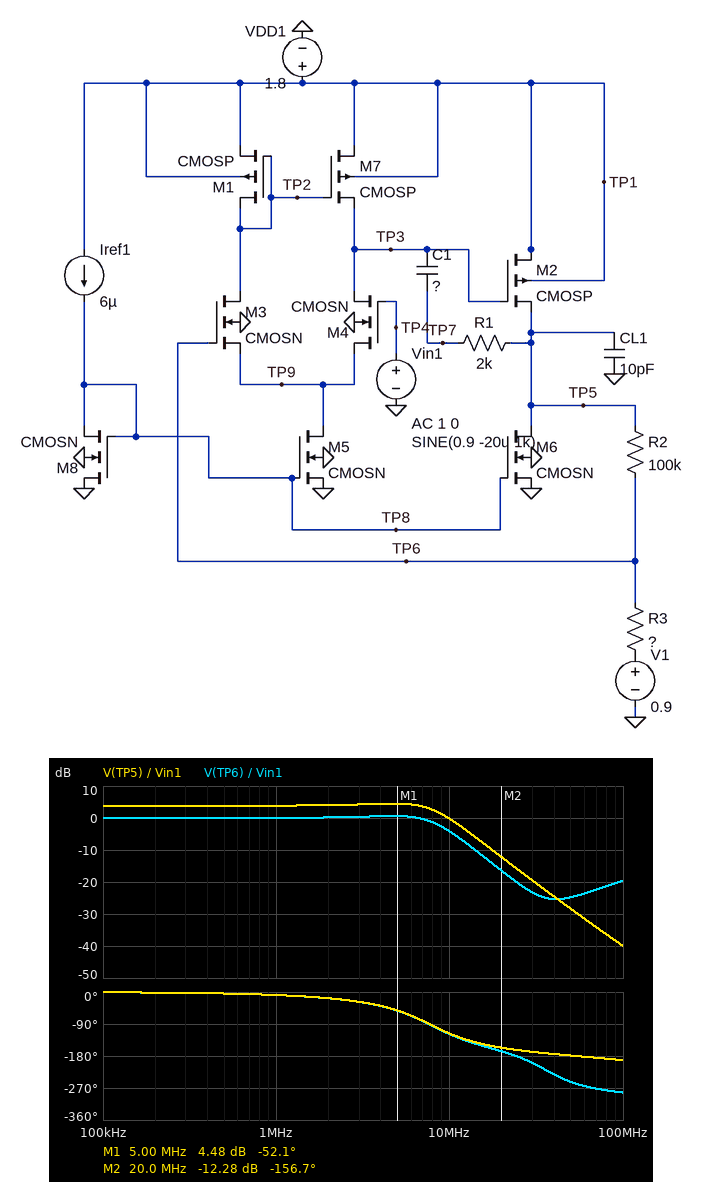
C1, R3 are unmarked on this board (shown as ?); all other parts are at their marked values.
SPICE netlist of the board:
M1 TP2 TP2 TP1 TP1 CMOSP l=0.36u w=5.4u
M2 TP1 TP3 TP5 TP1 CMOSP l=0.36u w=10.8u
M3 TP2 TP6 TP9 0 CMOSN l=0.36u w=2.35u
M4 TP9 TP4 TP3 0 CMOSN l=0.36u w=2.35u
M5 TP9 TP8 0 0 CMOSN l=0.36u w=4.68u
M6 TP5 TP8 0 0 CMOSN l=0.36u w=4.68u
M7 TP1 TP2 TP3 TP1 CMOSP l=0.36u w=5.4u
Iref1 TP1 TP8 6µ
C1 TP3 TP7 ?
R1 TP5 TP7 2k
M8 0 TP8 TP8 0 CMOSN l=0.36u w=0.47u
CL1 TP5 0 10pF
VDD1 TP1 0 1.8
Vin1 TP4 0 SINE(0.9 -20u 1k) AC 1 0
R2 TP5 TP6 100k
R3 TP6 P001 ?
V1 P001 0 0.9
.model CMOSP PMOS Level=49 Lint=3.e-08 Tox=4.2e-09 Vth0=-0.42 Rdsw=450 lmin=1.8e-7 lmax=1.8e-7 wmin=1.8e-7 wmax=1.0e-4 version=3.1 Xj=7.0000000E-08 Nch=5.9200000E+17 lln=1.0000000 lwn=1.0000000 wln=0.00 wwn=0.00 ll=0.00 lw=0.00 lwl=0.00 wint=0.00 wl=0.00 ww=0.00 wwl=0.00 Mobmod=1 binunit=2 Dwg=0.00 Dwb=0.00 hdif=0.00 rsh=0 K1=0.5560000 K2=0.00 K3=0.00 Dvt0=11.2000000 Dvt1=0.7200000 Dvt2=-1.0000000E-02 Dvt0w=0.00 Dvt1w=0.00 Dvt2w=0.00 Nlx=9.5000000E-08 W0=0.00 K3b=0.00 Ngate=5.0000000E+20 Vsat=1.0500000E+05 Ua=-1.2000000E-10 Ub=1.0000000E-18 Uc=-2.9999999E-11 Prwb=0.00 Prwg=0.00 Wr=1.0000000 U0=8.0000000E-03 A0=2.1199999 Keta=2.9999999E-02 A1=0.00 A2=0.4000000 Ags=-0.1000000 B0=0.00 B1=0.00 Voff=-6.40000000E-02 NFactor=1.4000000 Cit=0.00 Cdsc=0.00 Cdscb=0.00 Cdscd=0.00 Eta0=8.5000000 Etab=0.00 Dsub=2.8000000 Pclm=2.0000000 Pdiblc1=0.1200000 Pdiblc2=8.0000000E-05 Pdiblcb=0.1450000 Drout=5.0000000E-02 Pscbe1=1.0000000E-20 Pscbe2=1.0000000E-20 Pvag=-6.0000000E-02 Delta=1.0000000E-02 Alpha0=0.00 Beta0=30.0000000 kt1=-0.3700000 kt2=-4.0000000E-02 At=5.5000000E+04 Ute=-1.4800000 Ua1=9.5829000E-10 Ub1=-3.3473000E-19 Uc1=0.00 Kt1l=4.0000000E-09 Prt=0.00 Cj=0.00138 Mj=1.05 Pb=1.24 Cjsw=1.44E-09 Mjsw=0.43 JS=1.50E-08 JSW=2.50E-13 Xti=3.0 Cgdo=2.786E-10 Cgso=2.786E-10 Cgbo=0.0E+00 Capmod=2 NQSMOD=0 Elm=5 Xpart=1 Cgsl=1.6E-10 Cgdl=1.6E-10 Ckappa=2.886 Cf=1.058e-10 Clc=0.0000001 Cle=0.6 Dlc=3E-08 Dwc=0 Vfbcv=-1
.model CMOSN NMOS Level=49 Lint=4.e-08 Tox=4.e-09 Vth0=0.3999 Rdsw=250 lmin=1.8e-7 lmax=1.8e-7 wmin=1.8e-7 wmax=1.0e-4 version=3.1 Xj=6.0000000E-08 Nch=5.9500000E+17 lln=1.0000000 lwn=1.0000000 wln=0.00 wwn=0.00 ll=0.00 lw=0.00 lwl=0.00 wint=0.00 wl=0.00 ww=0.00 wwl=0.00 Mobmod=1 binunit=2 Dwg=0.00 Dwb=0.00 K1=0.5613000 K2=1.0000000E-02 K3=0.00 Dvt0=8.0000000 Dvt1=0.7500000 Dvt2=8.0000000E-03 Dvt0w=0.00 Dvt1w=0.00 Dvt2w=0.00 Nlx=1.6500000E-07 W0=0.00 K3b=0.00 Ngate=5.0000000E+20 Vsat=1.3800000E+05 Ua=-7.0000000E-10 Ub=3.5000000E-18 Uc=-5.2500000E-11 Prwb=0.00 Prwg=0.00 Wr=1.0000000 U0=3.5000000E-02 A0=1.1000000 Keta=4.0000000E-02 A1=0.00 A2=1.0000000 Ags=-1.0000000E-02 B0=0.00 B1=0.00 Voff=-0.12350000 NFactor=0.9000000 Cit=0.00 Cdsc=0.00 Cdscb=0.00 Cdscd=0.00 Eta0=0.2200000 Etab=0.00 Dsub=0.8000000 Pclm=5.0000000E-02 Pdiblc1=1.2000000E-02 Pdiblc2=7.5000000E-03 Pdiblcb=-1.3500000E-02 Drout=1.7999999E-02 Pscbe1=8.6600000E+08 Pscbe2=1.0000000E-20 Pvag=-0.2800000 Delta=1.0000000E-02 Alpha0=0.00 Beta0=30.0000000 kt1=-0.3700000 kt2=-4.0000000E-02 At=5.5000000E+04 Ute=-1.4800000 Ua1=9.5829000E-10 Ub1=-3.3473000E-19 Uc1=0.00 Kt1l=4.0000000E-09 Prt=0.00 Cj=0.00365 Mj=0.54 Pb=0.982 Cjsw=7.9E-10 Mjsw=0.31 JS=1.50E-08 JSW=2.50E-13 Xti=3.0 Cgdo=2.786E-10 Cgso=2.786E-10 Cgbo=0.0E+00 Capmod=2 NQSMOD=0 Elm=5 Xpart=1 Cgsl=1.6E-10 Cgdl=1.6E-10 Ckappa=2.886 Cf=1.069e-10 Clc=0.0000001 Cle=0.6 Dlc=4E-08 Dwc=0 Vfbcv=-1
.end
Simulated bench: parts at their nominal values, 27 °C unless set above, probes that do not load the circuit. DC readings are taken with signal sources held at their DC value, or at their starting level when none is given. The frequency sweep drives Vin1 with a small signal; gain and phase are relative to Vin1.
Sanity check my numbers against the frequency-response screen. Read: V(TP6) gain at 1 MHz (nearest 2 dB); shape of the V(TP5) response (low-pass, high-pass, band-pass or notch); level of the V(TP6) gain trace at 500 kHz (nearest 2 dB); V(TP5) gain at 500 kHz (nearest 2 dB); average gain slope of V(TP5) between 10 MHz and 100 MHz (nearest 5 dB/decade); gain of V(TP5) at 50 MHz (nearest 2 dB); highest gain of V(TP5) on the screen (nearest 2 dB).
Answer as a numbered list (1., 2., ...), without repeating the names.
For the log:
1. 0 dB
2. low-pass
3. 0 dB
4. 4 dB
5. -40 dB/decade
6. -28 dB
7. 4 dB
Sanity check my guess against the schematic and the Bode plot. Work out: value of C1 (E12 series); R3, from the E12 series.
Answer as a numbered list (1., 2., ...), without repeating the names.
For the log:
1. 3.3 pF
2. 180 kΩ
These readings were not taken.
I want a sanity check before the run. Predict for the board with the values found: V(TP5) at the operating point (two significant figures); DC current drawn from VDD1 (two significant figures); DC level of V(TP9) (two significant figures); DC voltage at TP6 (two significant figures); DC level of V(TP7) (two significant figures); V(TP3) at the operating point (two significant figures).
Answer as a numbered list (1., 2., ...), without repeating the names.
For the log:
1. 900 mV
2. 120 µA
3. 180 mV
4. 900 mV
5. 900 mV
6. 1.1 V
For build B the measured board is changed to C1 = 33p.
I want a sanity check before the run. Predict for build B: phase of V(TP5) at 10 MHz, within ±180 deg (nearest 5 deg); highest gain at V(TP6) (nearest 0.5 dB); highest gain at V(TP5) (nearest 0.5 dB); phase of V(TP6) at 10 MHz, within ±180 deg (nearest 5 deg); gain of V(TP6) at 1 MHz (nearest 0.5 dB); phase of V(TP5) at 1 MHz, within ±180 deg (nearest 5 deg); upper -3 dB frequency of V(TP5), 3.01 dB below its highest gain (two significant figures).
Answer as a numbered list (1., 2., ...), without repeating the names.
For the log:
1. -145 deg
2. 0 dB
3. 4.0 dB
4. -155 deg
5. -4.0 dB
6. -60 deg
7. 790 kHz
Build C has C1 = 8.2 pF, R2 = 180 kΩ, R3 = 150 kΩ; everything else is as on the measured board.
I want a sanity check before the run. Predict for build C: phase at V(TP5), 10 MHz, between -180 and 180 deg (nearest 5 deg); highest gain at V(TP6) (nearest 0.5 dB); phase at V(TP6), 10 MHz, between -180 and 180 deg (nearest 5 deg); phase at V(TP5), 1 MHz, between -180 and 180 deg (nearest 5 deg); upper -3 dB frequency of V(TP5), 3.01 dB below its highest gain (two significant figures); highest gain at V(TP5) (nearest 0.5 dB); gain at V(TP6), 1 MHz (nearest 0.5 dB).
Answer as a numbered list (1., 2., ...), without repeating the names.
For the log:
1. -135 deg
2. 0 dB
3. -145 deg
4. -30 deg
5. 2.6 MHz
6. 7.0 dB
7. -0.5 dB
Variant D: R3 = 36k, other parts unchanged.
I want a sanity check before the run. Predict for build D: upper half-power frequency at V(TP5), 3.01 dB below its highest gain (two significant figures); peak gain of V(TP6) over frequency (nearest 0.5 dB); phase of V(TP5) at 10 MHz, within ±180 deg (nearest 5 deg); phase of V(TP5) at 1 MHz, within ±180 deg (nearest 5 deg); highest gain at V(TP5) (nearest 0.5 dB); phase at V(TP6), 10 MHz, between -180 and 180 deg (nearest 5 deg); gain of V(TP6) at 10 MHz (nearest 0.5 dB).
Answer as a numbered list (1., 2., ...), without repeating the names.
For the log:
1. 3.8 MHz
2. 0 dB
3. -130 deg
4. -20 deg
5. 11.5 dB
6. -135 deg
7. -13.5 dB
